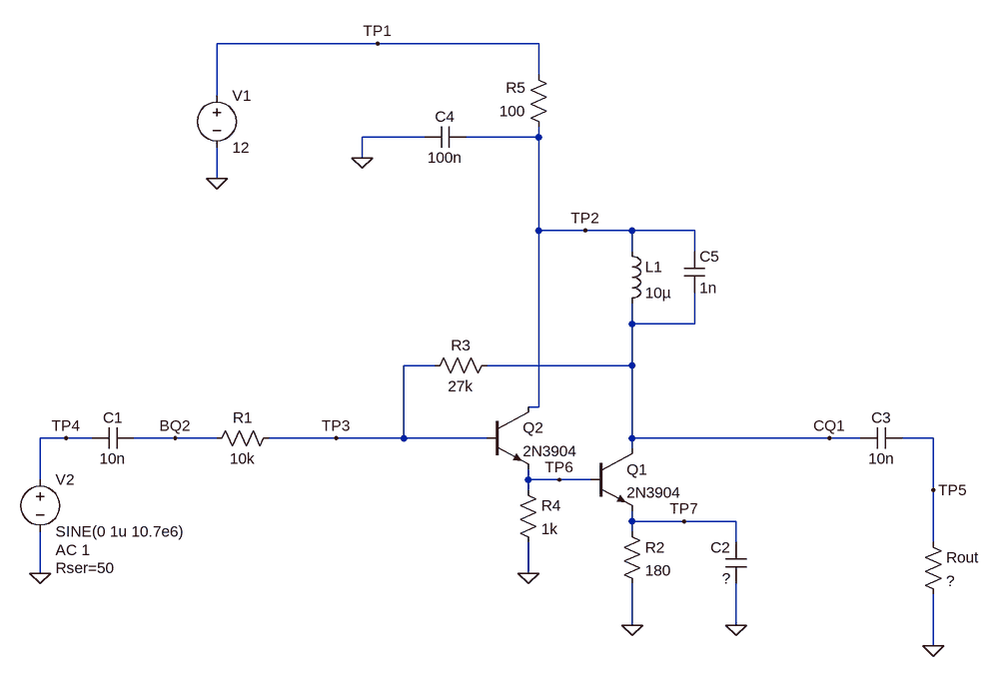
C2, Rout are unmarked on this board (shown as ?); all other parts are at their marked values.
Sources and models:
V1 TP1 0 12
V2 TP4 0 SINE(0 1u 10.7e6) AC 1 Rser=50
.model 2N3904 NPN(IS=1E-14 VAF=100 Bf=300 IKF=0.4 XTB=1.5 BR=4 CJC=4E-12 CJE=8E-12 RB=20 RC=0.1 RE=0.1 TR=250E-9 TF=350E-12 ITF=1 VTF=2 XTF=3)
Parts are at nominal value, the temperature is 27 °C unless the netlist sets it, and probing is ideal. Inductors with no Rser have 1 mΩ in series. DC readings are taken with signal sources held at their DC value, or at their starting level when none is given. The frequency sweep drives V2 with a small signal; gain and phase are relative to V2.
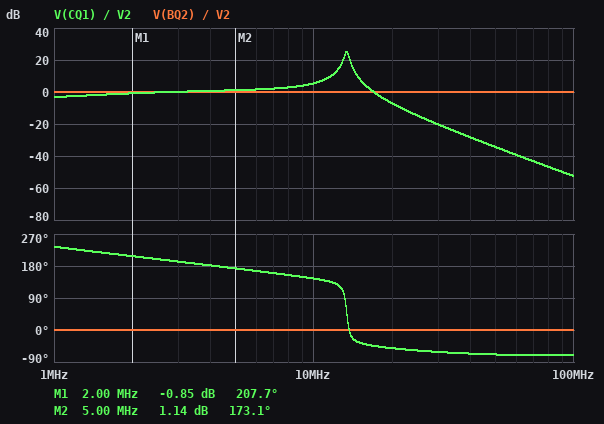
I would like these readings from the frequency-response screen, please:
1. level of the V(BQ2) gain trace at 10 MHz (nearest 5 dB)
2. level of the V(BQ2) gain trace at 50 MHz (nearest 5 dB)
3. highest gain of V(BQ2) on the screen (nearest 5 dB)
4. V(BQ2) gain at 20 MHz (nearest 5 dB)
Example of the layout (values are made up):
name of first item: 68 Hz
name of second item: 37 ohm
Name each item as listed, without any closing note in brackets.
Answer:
level of the V(BQ2) gain trace at 10 MHz: 0 dB
level of the V(BQ2) gain trace at 50 MHz: 0 dB
highest gain of V(BQ2) on the screen: 0 dB
V(BQ2) gain at 20 MHz: 0 dB
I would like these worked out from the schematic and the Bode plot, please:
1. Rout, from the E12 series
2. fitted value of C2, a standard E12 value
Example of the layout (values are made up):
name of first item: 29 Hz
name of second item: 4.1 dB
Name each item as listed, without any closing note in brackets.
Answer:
Rout, from the E12 series: 39 Ω
fitted value of C2, a standard E12 value: 3.9 nF
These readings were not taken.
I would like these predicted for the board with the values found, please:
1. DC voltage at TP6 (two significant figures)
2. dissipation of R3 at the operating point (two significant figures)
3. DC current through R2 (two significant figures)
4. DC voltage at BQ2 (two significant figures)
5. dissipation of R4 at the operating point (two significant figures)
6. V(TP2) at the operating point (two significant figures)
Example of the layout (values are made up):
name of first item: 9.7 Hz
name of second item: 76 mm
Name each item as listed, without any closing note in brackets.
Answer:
DC voltage at TP6: 6.7 V
dissipation of R3 at the operating point: 14 µW
DC current through R2: 33 mA
DC voltage at BQ2: 7.4 V
dissipation of R4 at the operating point: 45 mW
V(TP2) at the operating point: 8.0 V
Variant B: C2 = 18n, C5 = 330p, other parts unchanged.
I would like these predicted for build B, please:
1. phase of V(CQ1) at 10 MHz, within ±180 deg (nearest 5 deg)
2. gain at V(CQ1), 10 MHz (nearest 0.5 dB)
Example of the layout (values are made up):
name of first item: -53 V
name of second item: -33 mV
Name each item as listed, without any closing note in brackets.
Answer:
phase of V(CQ1) at 10 MHz, within ±180 deg: 160 deg
gain at V(CQ1), 10 MHz: 16.0 dB
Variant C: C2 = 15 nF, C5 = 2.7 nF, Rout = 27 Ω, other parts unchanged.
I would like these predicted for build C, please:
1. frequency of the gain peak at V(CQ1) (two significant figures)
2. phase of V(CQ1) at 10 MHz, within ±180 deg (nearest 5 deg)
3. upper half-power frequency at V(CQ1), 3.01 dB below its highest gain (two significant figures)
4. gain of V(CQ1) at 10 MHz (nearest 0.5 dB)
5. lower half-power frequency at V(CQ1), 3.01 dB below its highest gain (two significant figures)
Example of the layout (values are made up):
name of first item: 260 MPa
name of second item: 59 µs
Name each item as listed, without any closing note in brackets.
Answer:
frequency of the gain peak at V(CQ1): 8.3 MHz
phase of V(CQ1) at 10 MHz, within ±180 deg: -35 deg
upper half-power frequency at V(CQ1), 3.01 dB below its highest gain: 8.6 MHz
gain of V(CQ1) at 10 MHz: 6.0 dB
lower half-power frequency at V(CQ1), 3.01 dB below its highest gain: 8.0 MHz
